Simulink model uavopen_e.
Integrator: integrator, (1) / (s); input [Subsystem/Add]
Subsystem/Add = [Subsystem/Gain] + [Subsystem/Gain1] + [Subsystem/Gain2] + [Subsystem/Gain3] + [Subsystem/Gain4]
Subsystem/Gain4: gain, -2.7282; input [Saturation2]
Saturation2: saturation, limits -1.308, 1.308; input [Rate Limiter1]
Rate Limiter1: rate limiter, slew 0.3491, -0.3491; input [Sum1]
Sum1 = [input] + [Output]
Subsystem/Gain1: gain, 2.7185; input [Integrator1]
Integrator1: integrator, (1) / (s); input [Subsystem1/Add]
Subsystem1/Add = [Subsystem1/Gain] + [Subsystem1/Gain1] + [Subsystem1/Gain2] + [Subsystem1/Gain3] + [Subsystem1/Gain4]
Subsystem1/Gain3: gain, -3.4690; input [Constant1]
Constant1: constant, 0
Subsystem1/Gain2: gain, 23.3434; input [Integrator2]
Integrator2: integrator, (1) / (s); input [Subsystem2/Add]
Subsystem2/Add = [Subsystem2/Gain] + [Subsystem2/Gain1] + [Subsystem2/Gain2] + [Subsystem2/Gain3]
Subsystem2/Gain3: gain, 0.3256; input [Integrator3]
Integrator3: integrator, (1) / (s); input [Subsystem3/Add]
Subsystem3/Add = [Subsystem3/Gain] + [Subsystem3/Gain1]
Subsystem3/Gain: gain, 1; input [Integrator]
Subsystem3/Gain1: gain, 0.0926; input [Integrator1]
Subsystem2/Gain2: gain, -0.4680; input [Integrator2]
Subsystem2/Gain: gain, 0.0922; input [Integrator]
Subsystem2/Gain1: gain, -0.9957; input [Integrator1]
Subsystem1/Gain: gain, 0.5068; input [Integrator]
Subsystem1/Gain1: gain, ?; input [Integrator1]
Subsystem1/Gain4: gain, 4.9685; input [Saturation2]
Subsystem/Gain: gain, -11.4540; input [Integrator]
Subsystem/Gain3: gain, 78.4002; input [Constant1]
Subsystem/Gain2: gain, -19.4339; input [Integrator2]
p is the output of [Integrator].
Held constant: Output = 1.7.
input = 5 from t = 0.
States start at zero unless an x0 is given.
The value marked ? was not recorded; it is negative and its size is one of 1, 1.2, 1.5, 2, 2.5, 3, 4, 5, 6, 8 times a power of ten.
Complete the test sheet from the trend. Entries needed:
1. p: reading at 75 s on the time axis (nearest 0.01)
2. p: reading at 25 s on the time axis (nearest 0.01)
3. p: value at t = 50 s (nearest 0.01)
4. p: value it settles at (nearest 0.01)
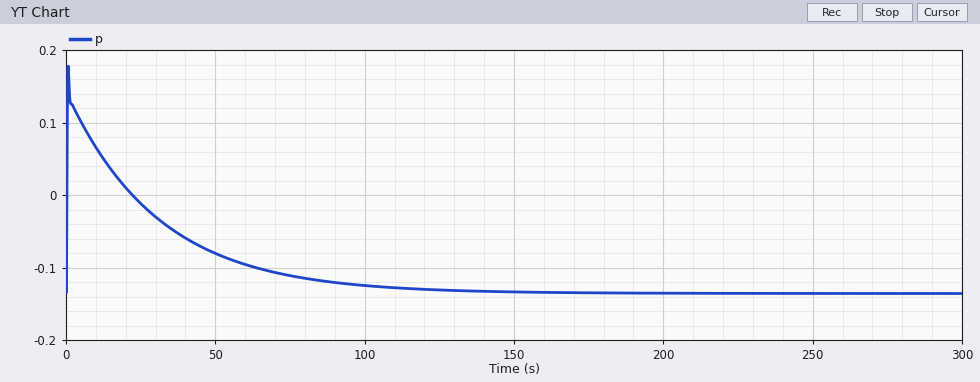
-0.11
-0.01
-0.08
-0.14
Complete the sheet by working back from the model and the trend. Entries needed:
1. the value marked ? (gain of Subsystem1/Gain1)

-6
